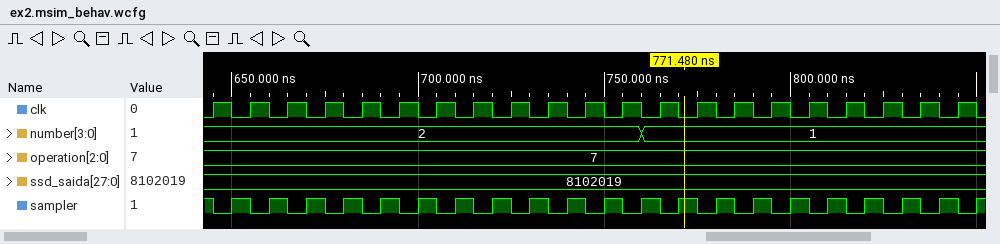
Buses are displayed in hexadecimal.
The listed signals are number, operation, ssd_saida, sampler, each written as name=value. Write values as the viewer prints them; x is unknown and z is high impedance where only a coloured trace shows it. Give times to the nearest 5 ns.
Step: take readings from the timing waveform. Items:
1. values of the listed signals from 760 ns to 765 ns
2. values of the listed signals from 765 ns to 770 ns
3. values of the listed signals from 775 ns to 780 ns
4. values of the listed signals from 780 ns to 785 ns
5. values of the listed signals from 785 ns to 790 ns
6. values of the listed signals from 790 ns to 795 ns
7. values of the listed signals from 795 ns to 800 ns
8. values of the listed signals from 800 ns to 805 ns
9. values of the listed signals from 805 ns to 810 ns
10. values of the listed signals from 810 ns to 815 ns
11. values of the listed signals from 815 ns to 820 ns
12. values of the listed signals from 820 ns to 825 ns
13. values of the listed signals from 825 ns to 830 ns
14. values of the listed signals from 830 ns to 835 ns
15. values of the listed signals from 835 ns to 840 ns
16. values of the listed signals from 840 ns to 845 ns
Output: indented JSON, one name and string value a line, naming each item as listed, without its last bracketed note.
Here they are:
{
  "values of the listed signals from 760 ns to 765 ns": "number=1, operation=7, ssd_saida=8102019, sampler=1",
  "values of the listed signals from 765 ns to 770 ns": "number=1, operation=7, ssd_saida=8102019, sampler=0",
  "values of the listed signals from 775 ns to 780 ns": "number=1, operation=7, ssd_saida=8102019, sampler=0",
  "values of the listed signals from 780 ns to 785 ns": "number=1, operation=7, ssd_saida=8102019, sampler=1",
  "values of the listed signals from 785 ns to 790 ns": "number=1, operation=7, ssd_saida=8102019, sampler=0",
  "values of the listed signals from 790 ns to 795 ns": "number=1, operation=7, ssd_saida=8102019, sampler=1",
  "values of the listed signals from 795 ns to 800 ns": "number=1, operation=7, ssd_saida=8102019, sampler=0",
  "values of the listed signals from 800 ns to 805 ns": "number=1, operation=7, ssd_saida=8102019, sampler=1",
  "values of the listed signals from 805 ns to 810 ns": "number=1, operation=7, ssd_saida=8102019, sampler=0",
  "values of the listed signals from 810 ns to 815 ns": "number=1, operation=7, ssd_saida=8102019, sampler=1",
  "values of the listed signals from 815 ns to 820 ns": "number=1, operation=7, ssd_saida=8102019, sampler=0",
  "values of the listed signals from 820 ns to 825 ns": "number=1, operation=7, ssd_saida=8102019, sampler=1",
  "values of the listed signals from 825 ns to 830 ns": "number=1, operation=7, ssd_saida=8102019, sampler=0",
  "values of the listed signals from 830 ns to 835 ns": "number=1, operation=7, ssd_saida=8102019, sampler=1",
  "values of the listed signals from 835 ns to 840 ns": "number=1, operation=7, ssd_saida=8102019, sampler=0",
  "values of the listed signals from 840 ns to 845 ns": "number=1, operation=7, ssd_saida=8102019, sampler=1"
}
